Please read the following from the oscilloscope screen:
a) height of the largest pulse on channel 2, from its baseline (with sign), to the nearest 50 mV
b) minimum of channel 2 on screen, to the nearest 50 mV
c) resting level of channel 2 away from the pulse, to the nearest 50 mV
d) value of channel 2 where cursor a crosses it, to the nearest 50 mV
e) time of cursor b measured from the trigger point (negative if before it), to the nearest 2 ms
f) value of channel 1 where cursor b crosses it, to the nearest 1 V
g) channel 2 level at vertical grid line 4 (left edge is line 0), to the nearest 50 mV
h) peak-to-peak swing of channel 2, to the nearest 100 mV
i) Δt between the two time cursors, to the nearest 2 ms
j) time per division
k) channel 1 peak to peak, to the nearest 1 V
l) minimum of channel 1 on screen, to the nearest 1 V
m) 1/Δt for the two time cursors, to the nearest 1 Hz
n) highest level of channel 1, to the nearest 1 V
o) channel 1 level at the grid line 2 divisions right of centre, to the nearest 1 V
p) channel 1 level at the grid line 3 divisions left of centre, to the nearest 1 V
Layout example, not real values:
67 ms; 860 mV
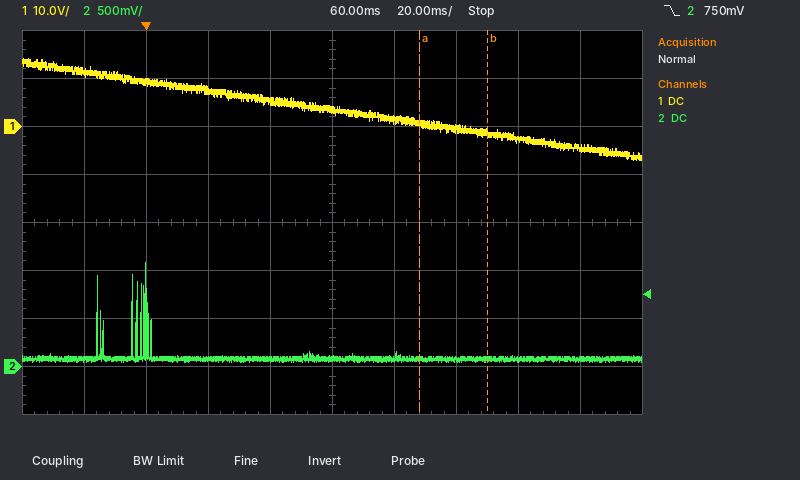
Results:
+1.00 V; 50 mV; 100 mV; 100 mV; +110 ms; -1 V; 100 mV; 1.00 V; 22 ms; 20 ms; 21 V; -7 V; 45 Hz; 14 V; 0 V; 9 V
